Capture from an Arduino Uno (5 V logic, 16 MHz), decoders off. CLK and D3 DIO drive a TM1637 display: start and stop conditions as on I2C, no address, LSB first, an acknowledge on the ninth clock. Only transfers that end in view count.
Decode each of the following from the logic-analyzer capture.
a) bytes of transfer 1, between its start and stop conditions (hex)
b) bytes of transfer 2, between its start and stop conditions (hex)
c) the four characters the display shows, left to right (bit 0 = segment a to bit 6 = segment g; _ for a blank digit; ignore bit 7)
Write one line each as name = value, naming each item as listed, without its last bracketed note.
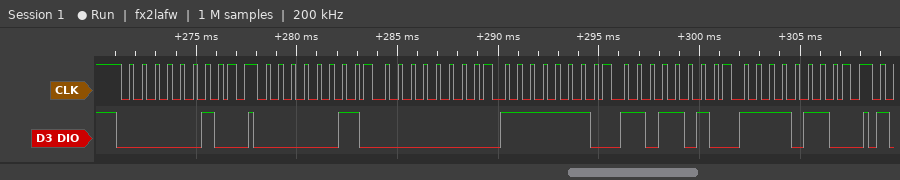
bytes of transfer 1, between its start and stop conditions = 40
bytes of transfer 2, between its start and stop conditions = C0 00 7F 5B 6F
the four characters the display shows, left to right = _829
